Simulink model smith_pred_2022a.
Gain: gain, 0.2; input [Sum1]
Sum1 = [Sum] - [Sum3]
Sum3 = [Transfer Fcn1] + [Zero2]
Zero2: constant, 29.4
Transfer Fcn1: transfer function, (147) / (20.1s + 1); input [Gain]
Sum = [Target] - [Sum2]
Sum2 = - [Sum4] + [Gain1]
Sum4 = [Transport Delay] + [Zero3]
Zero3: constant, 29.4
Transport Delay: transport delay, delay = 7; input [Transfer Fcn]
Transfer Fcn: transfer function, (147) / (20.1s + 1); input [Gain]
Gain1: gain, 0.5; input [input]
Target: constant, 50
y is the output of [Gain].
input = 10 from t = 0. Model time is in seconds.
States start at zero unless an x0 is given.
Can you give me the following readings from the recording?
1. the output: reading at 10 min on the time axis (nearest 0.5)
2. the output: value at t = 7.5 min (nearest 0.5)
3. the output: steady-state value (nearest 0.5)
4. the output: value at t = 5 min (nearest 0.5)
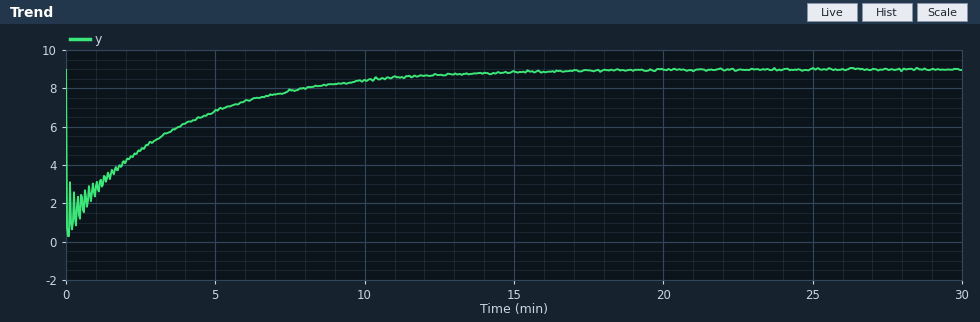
8.5
8.0
9.0
7.0
